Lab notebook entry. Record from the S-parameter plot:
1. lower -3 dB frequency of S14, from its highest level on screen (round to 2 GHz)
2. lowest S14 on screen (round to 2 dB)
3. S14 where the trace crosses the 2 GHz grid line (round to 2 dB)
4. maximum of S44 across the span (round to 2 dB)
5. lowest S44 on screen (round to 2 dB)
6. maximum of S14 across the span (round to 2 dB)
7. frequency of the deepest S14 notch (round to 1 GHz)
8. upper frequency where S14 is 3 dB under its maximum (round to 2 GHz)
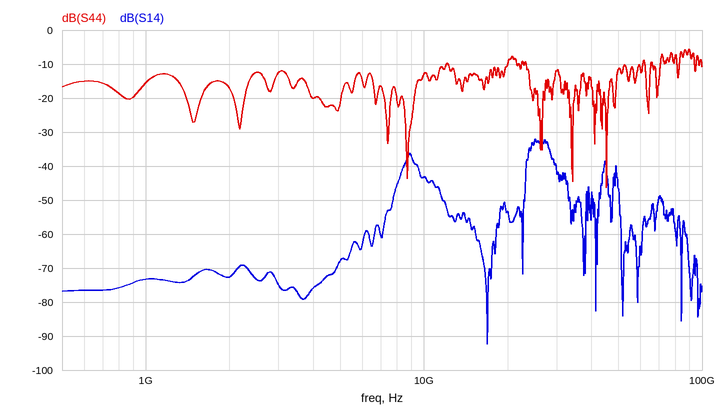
24 GHz
-92 dB
-72 dB
-6 dB
-46 dB
-32 dB
17 GHz
28 GHz
